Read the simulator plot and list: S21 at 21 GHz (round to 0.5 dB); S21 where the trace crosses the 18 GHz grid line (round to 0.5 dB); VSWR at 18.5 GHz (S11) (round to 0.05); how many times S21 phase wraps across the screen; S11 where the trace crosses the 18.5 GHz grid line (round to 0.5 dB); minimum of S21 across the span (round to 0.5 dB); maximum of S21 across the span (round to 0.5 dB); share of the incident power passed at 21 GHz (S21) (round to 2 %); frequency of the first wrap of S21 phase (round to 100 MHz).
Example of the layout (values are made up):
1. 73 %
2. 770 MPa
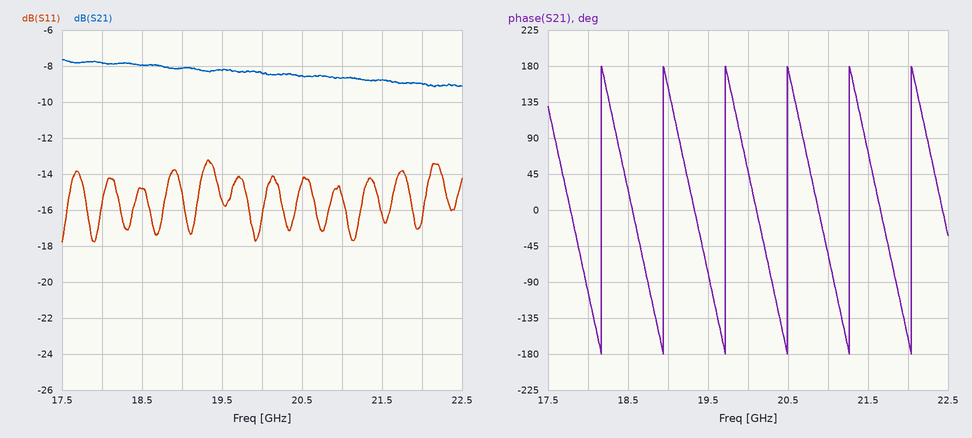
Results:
1. -8.5 dB
2. -8.0 dB
3. 1.45
4. 6
5. -15.0 dB
6. -9.0 dB
7. -7.5 dB
8. 14 %
9. 18.2 GHz
